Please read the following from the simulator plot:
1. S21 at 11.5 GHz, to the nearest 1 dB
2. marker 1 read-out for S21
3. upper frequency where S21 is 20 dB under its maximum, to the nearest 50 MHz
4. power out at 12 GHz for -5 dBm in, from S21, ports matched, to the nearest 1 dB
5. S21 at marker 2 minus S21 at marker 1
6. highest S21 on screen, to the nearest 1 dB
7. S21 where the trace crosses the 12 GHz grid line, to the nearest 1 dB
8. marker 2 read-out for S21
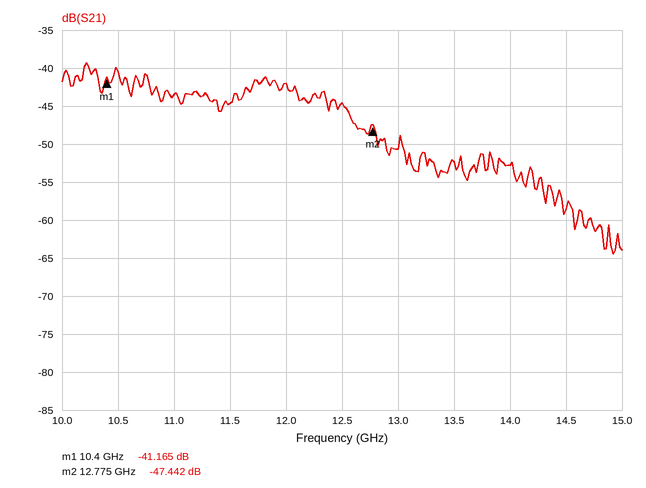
-45 dB
-41.165 dB
14.55 GHz
-47 dBm
-6.277 dB
-39 dB
-42 dB
-47.442 dB
